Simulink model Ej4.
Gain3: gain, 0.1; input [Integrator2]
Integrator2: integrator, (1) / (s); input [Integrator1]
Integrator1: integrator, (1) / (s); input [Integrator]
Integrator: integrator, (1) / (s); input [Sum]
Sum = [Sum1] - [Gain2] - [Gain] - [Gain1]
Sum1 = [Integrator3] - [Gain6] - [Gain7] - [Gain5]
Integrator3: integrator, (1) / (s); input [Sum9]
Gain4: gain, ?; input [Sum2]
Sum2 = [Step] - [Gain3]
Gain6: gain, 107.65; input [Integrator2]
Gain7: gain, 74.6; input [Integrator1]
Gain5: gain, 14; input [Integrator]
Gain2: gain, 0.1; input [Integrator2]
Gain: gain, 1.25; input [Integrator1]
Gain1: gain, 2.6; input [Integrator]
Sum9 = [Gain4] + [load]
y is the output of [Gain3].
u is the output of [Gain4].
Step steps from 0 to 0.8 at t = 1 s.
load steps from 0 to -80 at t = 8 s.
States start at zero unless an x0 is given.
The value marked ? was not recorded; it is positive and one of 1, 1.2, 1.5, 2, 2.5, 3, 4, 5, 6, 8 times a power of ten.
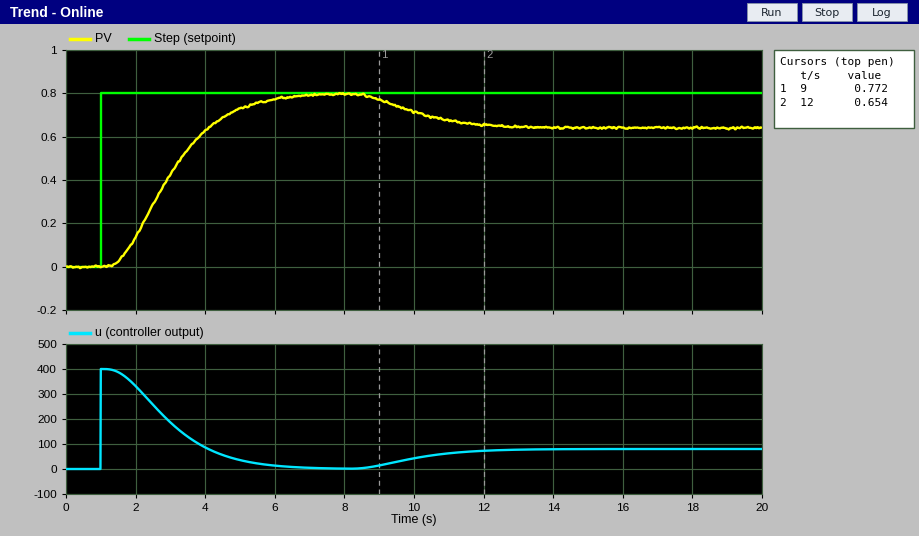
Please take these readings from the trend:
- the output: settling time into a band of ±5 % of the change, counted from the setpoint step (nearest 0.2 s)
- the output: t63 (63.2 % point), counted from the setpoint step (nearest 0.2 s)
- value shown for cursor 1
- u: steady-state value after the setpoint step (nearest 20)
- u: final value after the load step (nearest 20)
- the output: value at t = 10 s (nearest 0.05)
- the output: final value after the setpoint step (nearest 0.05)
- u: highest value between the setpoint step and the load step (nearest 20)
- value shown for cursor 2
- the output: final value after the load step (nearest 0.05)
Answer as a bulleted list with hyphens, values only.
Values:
- 4.6 s
- 2.4 s
- 0.772
- 0
- 80
- 0.70
- 0.80
- 400
- 0.654
- 0.65
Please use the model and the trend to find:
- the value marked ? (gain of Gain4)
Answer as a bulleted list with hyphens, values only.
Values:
- 500
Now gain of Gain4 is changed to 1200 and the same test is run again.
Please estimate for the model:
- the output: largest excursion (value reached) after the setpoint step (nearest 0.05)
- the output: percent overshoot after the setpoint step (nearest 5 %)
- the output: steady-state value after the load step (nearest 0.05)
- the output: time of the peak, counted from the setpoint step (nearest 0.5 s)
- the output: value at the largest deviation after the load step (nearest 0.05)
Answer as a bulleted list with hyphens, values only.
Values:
- 0.95
- 20 %
- 0.75
- 2.5 s
- 0.70
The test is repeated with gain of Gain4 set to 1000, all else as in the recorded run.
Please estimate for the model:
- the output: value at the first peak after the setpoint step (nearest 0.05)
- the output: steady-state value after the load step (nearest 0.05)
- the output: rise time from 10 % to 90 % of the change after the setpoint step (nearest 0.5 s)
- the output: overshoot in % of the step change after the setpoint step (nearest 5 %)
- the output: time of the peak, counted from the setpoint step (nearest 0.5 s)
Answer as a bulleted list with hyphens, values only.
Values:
- 0.90
- 0.70
- 1.5 s
- 10 %
- 3.0 s
